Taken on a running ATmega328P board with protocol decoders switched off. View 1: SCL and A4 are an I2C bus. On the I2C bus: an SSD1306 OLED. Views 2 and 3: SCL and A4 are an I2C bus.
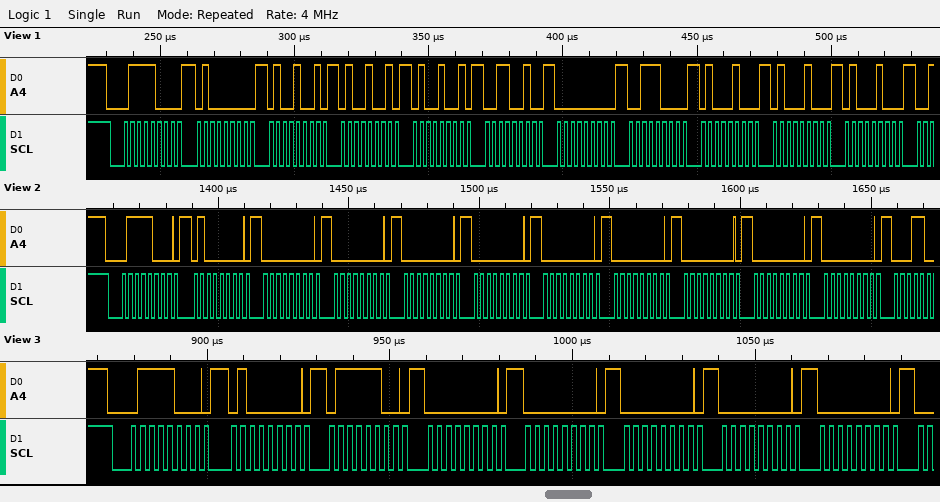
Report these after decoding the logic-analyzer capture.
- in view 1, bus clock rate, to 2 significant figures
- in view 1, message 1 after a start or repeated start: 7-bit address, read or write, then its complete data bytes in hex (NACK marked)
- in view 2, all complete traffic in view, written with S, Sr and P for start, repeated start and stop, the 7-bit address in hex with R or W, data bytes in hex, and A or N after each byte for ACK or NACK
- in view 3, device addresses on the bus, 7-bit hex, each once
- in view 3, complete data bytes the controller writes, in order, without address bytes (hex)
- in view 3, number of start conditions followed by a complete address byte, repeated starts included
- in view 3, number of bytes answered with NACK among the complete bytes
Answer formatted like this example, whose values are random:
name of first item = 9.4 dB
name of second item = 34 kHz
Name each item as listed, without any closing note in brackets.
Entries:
in view 1, bus clock rate, to 2 significant figures = 400 kHz
in view 1, message 1 after a start or repeated start: 7-bit address, read or write, then its complete data bytes in hex = 0x3C write: 40 49 49 49 32 00 38 44 44 44
in view 2, all complete traffic in view, written with S, Sr and P for start, repeated start and stop, the 7-bit address in hex with R or W, data bytes in hex, and A or N after each byte for ACK or NACK = S 3CW A 40 A 00 A 00 A 00 A 00 A 00 A 00 A 00 A 00 A 00 A
in view 3, device addresses on the bus, 7-bit hex, each once = 0x3C
in view 3, complete data bytes the controller writes, in order, without address bytes = 40 7C 00 00 00 00 00
in view 3, number of start conditions followed by a complete address byte, repeated starts included = 1
in view 3, number of bytes answered with NACK among the complete bytes = 0
